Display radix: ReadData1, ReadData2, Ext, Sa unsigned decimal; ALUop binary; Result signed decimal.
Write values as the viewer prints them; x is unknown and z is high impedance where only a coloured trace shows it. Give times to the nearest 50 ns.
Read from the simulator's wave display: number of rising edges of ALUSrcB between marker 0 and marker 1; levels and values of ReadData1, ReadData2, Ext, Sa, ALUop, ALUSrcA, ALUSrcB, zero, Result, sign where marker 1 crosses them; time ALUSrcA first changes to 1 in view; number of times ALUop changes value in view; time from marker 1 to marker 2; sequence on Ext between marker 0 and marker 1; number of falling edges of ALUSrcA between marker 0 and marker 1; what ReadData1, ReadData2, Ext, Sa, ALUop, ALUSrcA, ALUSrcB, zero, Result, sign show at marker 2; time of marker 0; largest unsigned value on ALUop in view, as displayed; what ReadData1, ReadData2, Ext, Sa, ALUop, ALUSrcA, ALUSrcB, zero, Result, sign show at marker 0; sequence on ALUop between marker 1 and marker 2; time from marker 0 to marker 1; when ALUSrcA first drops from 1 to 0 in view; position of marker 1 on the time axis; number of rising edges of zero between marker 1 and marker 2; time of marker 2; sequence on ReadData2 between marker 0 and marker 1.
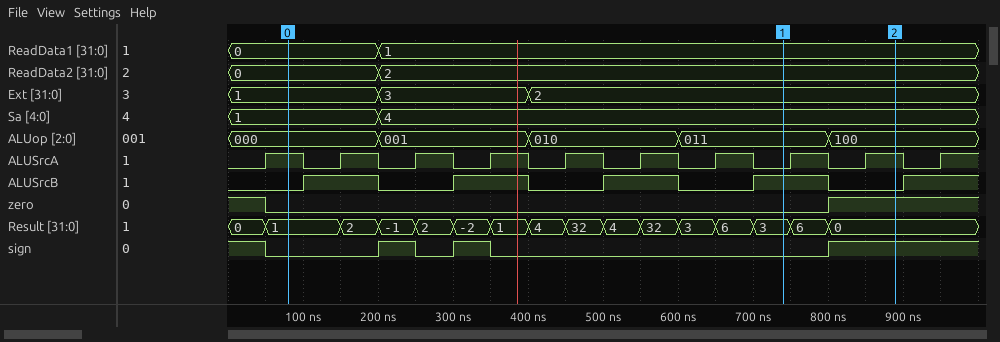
4
ReadData1=1, ReadData2=2, Ext=2, Sa=4, ALUop=011, ALUSrcA=0, ALUSrcB=1, zero=0, Result=3, sign=0
50 ns
4
150 ns
1, 3, 2
7
ReadData1=1, ReadData2=2, Ext=2, Sa=4, ALUop=100, ALUSrcA=1, ALUSrcB=0, zero=1, Result=0, sign=1
100 ns
100
ReadData1=0, ReadData2=0, Ext=1, Sa=1, ALUop=000, ALUSrcA=1, ALUSrcB=0, zero=0, Result=1, sign=0
011, 100
650 ns
100 ns
750 ns
1
900 ns
0, 2
